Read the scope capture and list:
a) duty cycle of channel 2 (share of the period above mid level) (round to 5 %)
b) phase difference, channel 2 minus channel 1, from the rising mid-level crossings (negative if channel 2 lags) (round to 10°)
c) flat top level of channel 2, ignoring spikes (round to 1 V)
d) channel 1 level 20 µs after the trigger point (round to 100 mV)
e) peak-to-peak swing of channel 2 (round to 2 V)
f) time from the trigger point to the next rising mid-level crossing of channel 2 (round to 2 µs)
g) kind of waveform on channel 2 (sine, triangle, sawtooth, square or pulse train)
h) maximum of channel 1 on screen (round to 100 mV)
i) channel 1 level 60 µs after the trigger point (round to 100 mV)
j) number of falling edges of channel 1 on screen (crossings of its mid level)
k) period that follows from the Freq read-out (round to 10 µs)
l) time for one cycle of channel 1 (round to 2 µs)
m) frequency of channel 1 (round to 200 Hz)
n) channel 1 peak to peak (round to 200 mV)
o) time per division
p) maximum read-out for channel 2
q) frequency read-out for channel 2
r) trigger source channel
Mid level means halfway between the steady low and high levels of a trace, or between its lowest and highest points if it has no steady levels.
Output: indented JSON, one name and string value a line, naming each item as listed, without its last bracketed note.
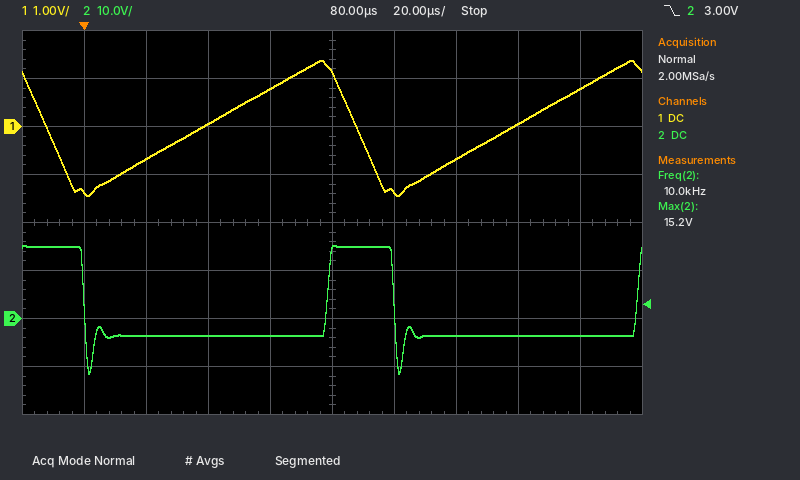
{
  "duty cycle of channel 2 (share of the period above mid level)": "20 %",
  "phase difference, channel 2 minus channel 1, from the rising mid-level crossings (negative if channel 2 lags)": "-150°",
  "flat top level of channel 2, ignoring spikes": "15 V",
  "channel 1 level 20 µs after the trigger point": "-700 mV",
  "peak-to-peak swing of channel 2": "26 V",
  "time from the trigger point to the next rising mid-level crossing of channel 2": "78 µs",
  "kind of waveform on channel 2": "pulse train",
  "maximum of channel 1 on screen": "1.4 V",
  "channel 1 level 60 µs after the trigger point": "800 mV",
  "number of falling edges of channel 1 on screen": "2",
  "period that follows from the Freq read-out": "100 µs",
  "time for one cycle of channel 1": "100 µs",
  "frequency of channel 1": "10.0 kHz",
  "channel 1 peak to peak": "2.8 V",
  "time per division": "20 µs",
  "maximum read-out for channel 2": "15.2 V",
  "frequency read-out for channel 2": "10.0 kHz",
  "trigger source channel": "channel 2"
}
